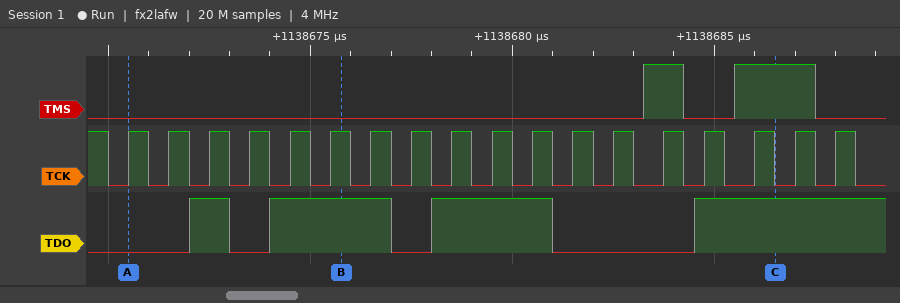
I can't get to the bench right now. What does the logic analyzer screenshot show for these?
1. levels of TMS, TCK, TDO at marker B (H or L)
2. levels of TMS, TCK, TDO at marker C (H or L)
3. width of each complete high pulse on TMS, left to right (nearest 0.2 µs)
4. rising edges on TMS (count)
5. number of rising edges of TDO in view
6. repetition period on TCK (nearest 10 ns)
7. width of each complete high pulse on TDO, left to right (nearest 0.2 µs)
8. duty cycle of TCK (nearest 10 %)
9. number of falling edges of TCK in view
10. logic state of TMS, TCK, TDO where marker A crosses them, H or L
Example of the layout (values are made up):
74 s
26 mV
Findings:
TMS=L, TCK=H, TDO=H
TMS=H, TCK=L, TDO=H
1 µs, 2 µs
2
4
1030 ns
1 µs, 3 µs, 3 µs
50 %
19
TMS=L, TCK=H, TDO=L
